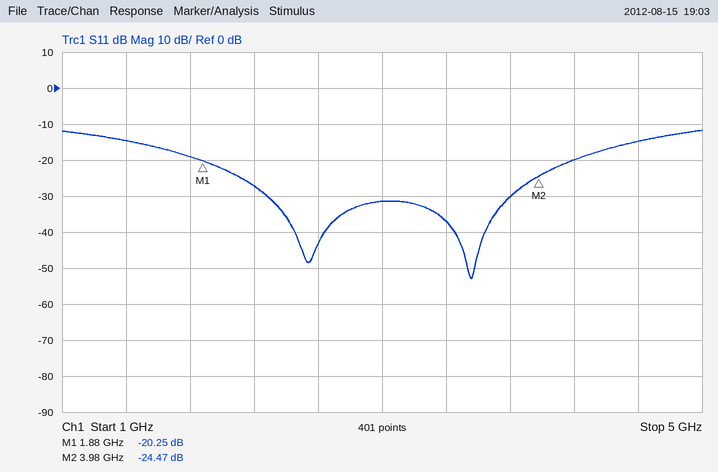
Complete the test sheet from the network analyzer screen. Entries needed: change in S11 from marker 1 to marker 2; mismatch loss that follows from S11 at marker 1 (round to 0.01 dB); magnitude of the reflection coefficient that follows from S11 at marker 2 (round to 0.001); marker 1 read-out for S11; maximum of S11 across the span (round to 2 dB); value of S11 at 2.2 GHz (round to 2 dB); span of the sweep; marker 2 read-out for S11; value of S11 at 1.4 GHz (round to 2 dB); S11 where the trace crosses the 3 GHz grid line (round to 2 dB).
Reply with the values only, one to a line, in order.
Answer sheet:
-4.22 dB
0.04 dB
0.060
-20.25 dB
-12 dB
-28 dB
4 GHz
-24.47 dB
-14 dB
-32 dB
